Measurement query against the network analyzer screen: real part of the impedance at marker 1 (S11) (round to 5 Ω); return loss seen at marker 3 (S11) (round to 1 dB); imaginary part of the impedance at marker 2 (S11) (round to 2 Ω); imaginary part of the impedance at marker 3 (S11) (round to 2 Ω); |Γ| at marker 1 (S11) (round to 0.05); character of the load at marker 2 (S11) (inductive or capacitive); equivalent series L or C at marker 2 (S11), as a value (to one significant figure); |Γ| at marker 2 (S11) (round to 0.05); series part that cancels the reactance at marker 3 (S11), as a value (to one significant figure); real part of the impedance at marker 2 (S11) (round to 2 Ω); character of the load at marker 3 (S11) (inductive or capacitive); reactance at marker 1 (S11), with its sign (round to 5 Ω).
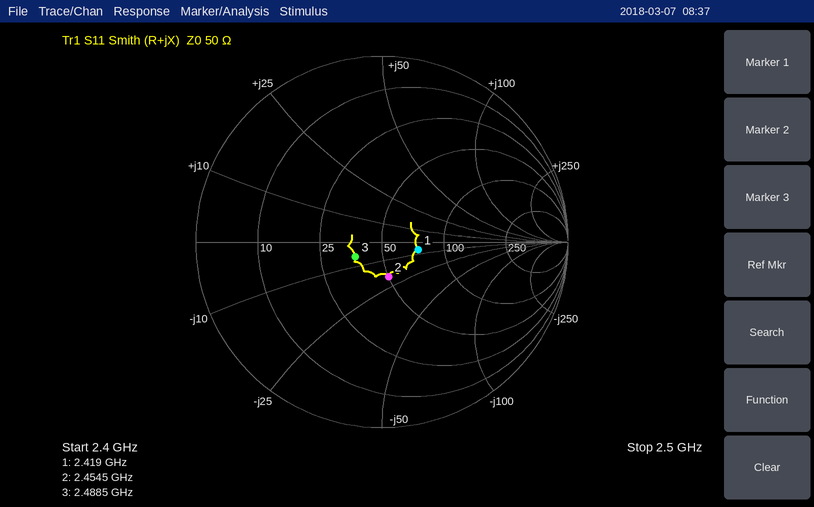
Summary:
75 Ω
16 dB
-20 Ω
-6 Ω
0.20
capacitive
3 pF
0.20
400 pH
50 Ω
capacitive
-5 Ω
